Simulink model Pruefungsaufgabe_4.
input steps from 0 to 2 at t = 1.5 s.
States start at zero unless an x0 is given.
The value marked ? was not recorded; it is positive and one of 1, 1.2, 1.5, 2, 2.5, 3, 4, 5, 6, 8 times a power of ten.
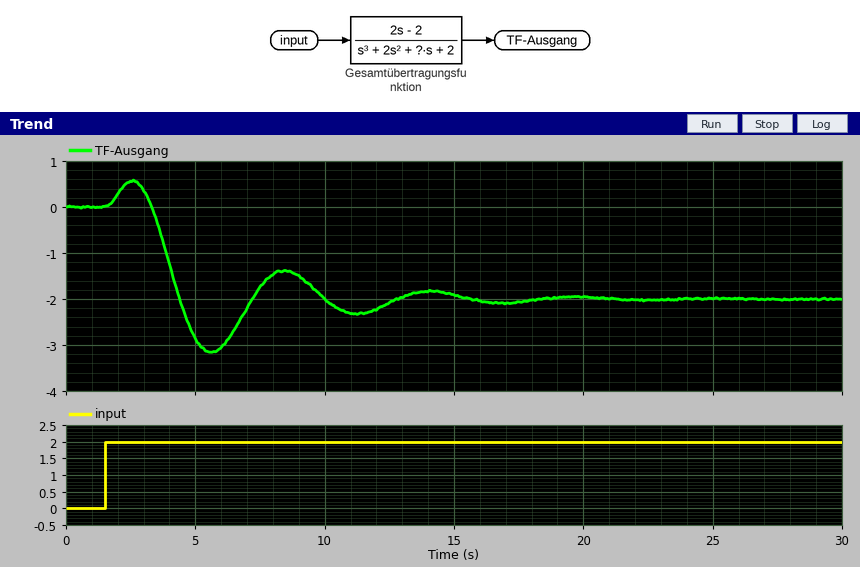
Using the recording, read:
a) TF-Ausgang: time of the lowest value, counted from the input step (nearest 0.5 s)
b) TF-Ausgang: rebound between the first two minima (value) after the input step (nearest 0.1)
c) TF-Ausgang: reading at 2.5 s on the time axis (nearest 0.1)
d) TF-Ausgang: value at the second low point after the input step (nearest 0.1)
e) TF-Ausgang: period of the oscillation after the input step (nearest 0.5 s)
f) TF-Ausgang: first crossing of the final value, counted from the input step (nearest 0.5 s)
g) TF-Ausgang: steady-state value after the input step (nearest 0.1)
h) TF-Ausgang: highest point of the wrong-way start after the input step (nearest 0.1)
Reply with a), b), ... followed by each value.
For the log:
a) 4.0 s
b) -1.4
c) 0.6
d) -2.3
e) 5.5 s
f) 3.0 s
g) -2.0
h) 0.6
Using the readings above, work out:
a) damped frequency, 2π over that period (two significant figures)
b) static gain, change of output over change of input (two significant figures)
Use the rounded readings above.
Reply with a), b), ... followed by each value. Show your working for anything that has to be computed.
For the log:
a) 2π / 5.5 = 1.1 rad/s
b) (-2 - 0) / (2 - 0) = -1.0
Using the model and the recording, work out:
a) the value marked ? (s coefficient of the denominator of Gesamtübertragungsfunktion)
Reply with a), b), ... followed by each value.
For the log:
a) 2
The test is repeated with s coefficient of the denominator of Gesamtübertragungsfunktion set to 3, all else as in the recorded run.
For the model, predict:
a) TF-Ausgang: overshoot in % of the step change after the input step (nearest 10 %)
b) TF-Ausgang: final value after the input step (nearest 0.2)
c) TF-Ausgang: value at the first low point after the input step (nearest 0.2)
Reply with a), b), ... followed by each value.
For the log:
a) 20 %
b) -2.0
c) -2.4
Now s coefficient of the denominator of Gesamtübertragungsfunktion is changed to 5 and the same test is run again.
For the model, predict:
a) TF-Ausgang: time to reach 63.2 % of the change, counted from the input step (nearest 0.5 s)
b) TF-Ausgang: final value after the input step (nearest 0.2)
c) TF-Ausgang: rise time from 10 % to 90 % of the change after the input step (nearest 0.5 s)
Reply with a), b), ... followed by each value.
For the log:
a) 3.0 s
b) -2.0
c) 4.0 s
